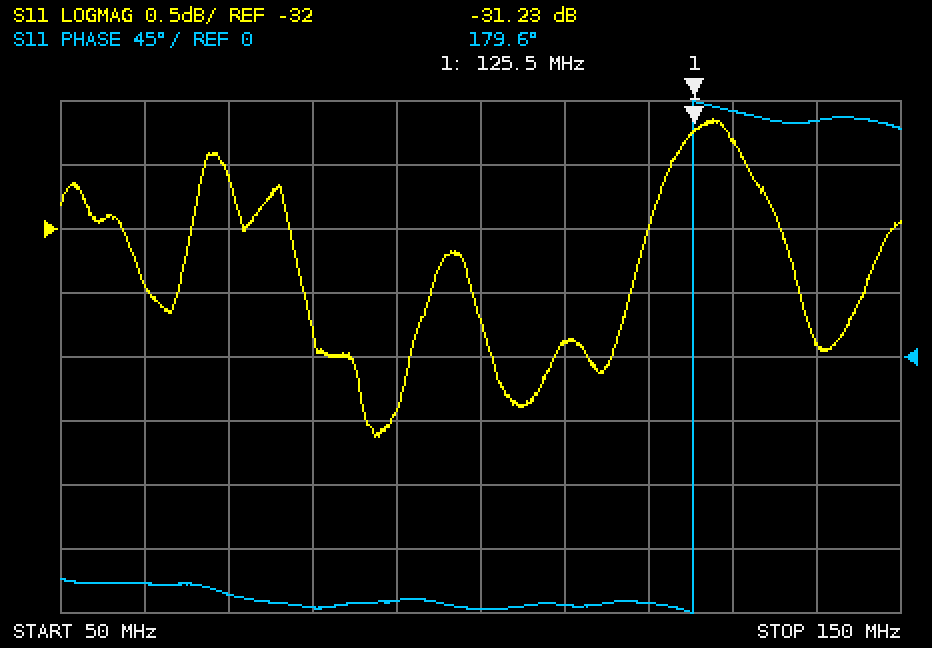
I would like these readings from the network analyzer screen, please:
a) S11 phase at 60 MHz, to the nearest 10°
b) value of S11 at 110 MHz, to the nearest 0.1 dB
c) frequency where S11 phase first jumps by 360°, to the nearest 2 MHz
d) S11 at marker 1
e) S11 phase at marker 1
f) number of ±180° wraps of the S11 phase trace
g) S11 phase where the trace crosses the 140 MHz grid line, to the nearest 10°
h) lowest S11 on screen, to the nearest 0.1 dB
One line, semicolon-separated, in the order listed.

-160°; -32.9 dB; 126 MHz; -31.23 dB; 179.6°; 1; 170°; -33.6 dB
